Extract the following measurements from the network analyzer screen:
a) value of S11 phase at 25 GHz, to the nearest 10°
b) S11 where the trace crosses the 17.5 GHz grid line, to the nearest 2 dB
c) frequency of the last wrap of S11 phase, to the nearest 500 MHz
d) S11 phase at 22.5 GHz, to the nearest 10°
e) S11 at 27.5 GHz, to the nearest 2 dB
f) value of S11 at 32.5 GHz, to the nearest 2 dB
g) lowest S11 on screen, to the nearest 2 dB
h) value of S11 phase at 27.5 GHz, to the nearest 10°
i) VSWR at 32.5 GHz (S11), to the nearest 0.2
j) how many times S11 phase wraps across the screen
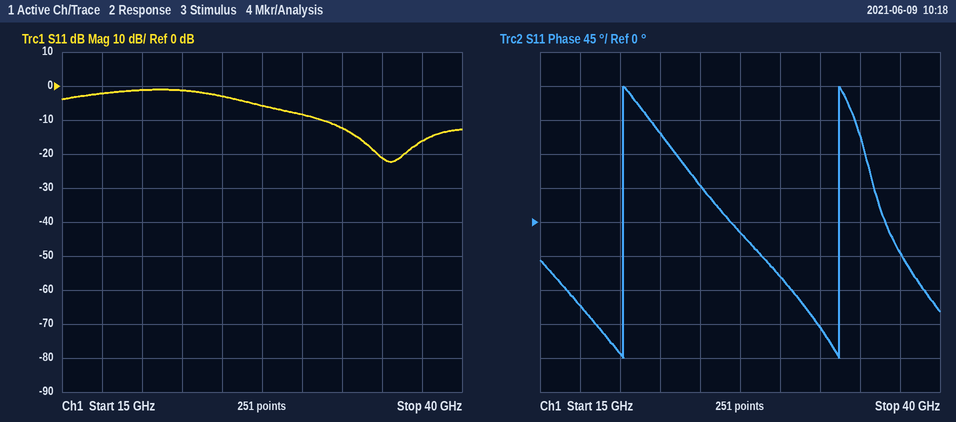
50°
-2 dB
33.5 GHz
120°
-6 dB
-12 dB
-22 dB
-10°
1.6
2
